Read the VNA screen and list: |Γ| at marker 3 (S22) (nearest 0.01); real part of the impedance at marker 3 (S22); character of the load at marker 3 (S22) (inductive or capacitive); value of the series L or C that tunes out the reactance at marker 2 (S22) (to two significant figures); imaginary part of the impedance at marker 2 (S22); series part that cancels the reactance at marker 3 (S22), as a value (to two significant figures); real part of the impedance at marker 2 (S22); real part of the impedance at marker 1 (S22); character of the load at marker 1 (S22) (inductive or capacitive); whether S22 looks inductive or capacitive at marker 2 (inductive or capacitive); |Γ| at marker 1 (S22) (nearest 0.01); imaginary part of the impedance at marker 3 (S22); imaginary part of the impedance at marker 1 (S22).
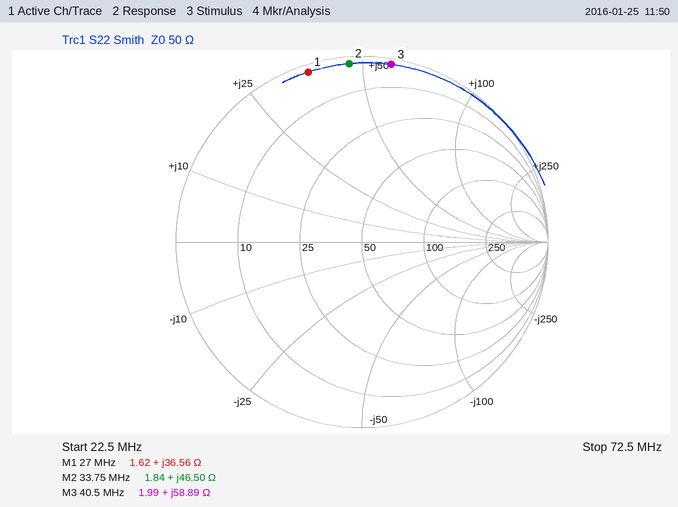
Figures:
0.97
1.99 Ω
inductive
100 pF
+46.50 Ω
67 pF
1.84 Ω
1.62 Ω
inductive
inductive
0.96
+58.89 Ω
+36.56 Ω
